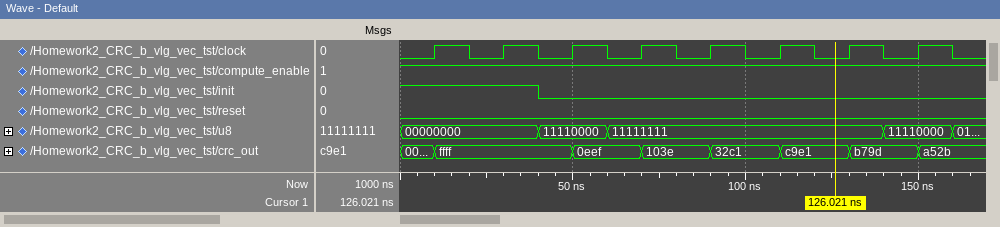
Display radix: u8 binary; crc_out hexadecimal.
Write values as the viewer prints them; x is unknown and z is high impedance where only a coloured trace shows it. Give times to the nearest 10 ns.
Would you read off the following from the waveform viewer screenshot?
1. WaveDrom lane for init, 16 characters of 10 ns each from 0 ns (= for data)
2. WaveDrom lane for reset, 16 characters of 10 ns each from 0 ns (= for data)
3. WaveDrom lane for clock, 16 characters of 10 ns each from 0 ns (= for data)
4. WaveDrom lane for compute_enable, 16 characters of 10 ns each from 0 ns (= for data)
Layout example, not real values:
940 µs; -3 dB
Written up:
{name: 'init', wave: '1...0...........'}; {name: 'reset', wave: '0...............'}; {name: 'clock', wave: '0101010101010101'}; {name: 'compute_enable', wave: '1...............'}
